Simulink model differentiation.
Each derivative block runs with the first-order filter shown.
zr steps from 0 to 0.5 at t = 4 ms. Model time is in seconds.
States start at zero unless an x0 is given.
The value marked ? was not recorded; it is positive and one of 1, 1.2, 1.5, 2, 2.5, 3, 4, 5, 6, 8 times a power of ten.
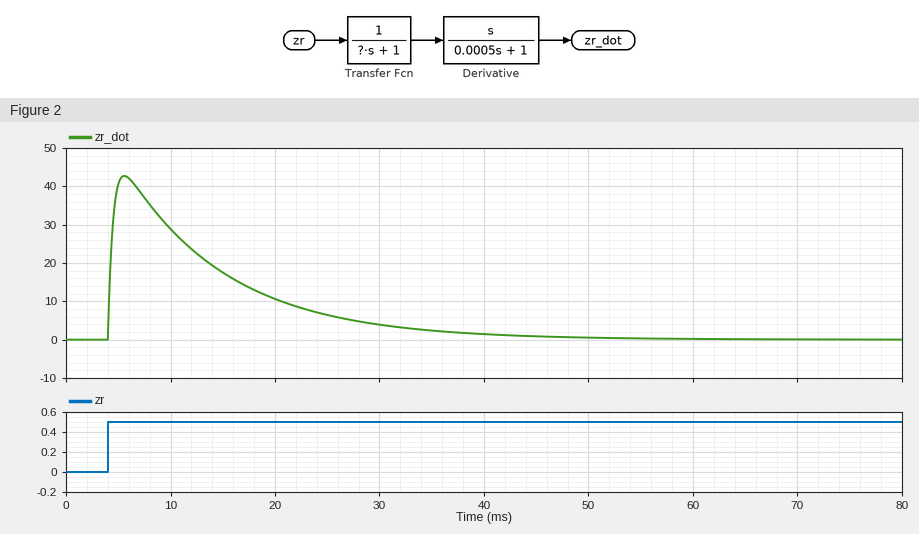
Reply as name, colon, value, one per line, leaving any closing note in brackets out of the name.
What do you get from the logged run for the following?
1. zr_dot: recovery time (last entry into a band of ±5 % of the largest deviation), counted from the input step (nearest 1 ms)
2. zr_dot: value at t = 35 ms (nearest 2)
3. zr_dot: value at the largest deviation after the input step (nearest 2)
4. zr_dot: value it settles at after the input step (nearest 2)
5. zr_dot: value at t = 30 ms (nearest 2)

zr_dot: recovery time (last entry into a band of ±5 % of the largest deviation), counted from the input step: 32 ms
zr_dot: value at t = 35 ms: 2
zr_dot: value at the largest deviation after the input step: 42
zr_dot: value it settles at after the input step: 0
zr_dot: value at t = 30 ms: 4
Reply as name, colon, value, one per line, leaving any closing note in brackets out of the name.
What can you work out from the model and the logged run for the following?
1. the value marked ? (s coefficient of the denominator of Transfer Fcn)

the value marked ?: 0.01
